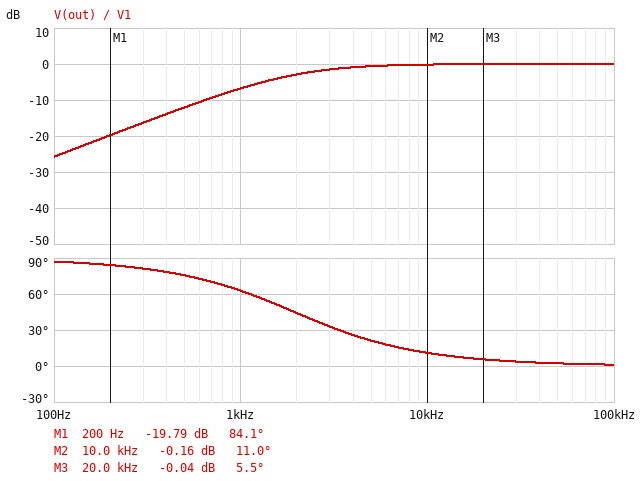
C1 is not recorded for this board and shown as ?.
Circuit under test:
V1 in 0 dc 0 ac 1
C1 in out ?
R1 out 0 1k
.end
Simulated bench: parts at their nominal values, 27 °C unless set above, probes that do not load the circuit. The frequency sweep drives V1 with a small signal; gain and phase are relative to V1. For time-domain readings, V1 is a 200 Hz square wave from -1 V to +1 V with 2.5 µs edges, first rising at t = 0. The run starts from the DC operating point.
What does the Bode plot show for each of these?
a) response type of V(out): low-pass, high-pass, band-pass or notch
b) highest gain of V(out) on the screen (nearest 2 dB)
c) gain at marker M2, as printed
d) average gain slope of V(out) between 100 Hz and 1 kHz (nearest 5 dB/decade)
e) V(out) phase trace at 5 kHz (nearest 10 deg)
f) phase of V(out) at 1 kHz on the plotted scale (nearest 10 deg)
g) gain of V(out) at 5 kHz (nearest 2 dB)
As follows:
high-pass
0 dB
-0.16 dB
20 dB/decade
20 deg
60 deg
0 dB
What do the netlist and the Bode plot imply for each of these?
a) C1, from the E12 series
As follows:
82 nF
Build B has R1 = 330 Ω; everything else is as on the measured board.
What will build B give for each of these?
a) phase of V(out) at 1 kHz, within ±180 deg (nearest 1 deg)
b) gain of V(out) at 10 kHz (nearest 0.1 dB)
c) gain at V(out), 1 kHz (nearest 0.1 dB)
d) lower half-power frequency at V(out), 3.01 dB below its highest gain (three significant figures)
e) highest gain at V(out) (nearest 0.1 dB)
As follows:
80 deg
-1.3 dB
-15.5 dB
5.88 kHz
0 dB
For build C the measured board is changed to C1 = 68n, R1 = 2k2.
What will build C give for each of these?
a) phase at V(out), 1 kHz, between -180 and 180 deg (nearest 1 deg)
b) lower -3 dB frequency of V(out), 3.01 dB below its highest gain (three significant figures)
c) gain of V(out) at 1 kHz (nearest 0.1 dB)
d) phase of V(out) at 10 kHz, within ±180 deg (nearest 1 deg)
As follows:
47 deg
1.06 kHz
-3.3 dB
6 deg
